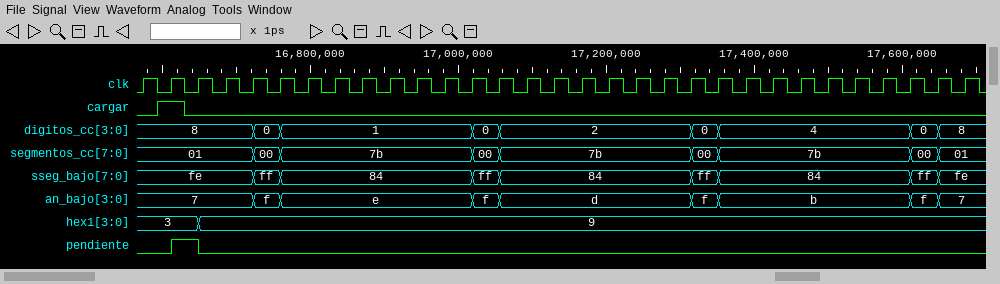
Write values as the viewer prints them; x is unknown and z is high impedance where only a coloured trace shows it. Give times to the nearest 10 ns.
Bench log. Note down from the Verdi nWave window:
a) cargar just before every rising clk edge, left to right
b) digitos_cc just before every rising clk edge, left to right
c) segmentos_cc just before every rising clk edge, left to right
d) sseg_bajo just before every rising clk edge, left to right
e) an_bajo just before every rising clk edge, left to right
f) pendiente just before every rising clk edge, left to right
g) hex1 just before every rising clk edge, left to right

0 1 0 0 0 0 0 0 0 0 0 0 0 0 0 0 0 0 0 0 0 0 0 0 0 0 0 0 0 0 0
8, 8, 8, 8, 8, 0, 1, 1, 1, 1, 1, 1, 1, 0, 2, 2, 2, 2, 2, 2, 2, 0, 4, 4, 4, 4, 4, 4, 4, 0, 8
01, 01, 01, 01, 01, 00, 7b, 7b, 7b, 7b, 7b, 7b, 7b, 00, 7b, 7b, 7b, 7b, 7b, 7b, 7b, 00, 7b, 7b, 7b, 7b, 7b, 7b, 7b, 00, 01
fe, fe, fe, fe, fe, ff, 84, 84, 84, 84, 84, 84, 84, ff, 84, 84, 84, 84, 84, 84, 84, ff, 84, 84, 84, 84, 84, 84, 84, ff, fe
7, 7, 7, 7, 7, f, e, e, e, e, e, e, e, f, d, d, d, d, d, d, d, f, b, b, b, b, b, b, b, f, 7
0 0 1 0 0 0 0 0 0 0 0 0 0 0 0 0 0 0 0 0 0 0 0 0 0 0 0 0 0 0 0
3, 3, 3, 9, 9, 9, 9, 9, 9, 9, 9, 9, 9, 9, 9, 9, 9, 9, 9, 9, 9, 9, 9, 9, 9, 9, 9, 9, 9, 9, 9
